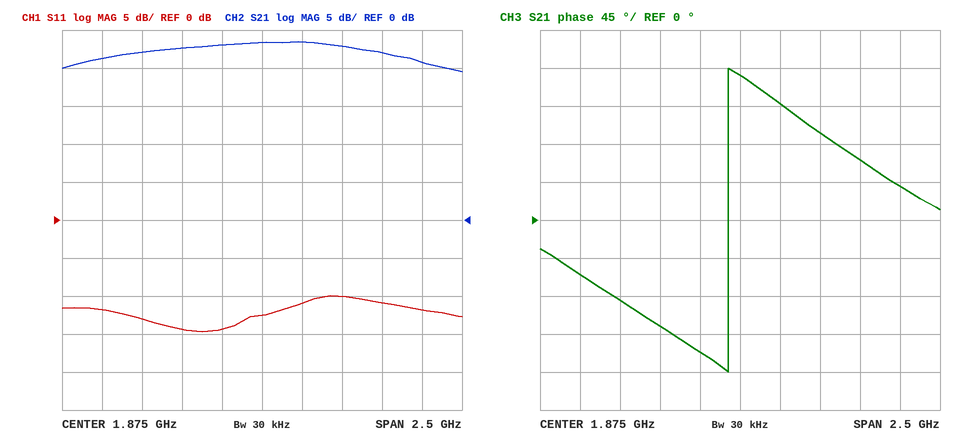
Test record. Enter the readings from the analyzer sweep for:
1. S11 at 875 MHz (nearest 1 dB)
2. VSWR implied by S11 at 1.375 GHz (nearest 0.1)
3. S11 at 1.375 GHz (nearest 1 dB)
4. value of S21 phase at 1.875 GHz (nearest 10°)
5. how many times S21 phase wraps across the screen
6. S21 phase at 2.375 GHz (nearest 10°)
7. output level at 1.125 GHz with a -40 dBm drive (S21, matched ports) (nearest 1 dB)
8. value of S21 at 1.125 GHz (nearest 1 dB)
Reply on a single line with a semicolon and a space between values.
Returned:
-12 dB; 1.5; -14 dB; 170°; 1; 100°; -18 dBm; 22 dB
